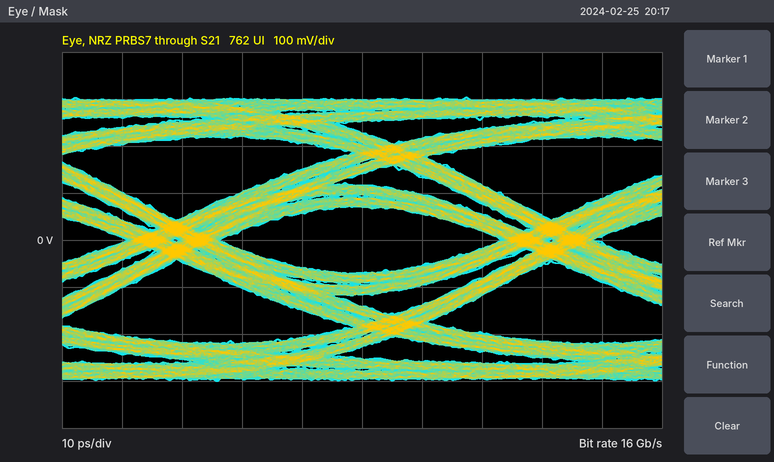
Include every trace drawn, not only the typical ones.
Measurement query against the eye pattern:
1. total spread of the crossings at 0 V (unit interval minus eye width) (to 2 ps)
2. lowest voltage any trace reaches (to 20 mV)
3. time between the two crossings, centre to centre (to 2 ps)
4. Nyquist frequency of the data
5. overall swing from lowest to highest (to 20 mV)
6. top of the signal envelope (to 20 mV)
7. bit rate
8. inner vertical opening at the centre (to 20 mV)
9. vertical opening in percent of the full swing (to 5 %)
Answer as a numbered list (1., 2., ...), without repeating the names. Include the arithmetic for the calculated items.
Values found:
1. 16 ps
2. -300 mV
3. 62 ps
4. 8 GHz
5. 600 mV
6. 300 mV
7. 16 Gb/s
8. 140 mV
9. 140 mV / 600 mV ≈ 23.3 %, so 25 % to the nearest 5 %
